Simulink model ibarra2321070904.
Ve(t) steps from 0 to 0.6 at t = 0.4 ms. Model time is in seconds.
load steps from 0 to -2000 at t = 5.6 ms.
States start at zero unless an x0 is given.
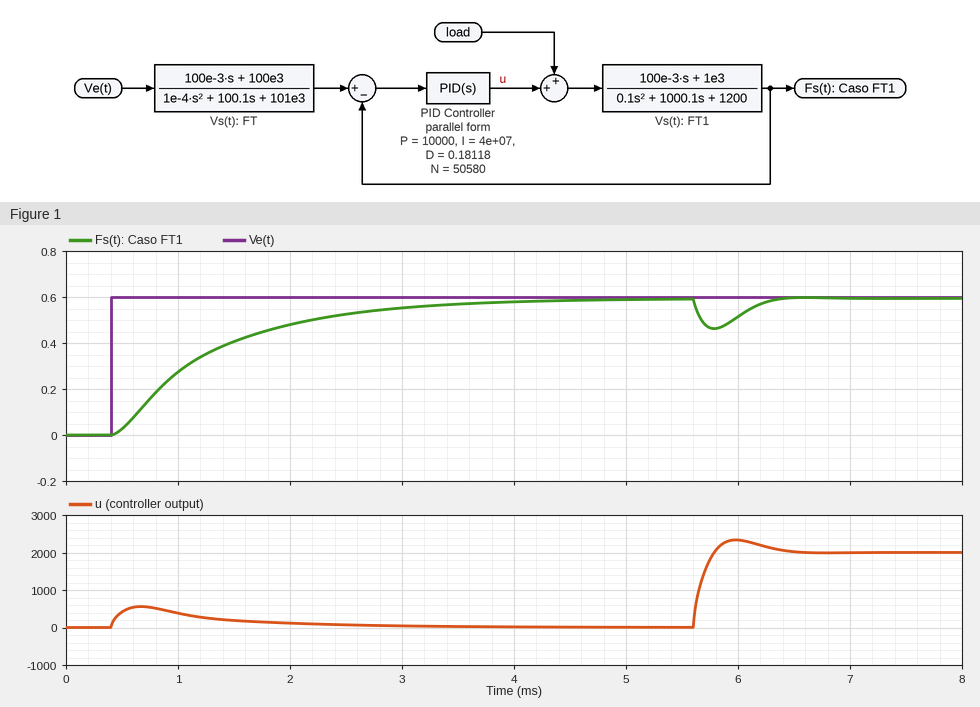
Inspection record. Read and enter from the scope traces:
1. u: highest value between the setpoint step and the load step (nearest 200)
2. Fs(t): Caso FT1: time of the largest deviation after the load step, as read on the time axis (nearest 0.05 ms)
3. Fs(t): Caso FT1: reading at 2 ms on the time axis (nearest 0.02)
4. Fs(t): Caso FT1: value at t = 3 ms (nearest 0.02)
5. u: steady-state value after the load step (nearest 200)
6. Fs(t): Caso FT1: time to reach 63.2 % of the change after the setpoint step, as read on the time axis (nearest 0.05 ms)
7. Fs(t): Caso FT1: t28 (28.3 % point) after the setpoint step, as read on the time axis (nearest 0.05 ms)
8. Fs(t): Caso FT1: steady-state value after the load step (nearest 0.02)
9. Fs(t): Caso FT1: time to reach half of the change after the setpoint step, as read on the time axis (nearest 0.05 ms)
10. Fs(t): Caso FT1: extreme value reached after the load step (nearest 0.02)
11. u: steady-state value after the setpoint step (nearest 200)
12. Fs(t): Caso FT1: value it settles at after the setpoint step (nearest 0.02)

600
5.80 ms
0.48
0.56
2000
1.35 ms
0.75 ms
0.60
1.05 ms
0.46
0
0.60
